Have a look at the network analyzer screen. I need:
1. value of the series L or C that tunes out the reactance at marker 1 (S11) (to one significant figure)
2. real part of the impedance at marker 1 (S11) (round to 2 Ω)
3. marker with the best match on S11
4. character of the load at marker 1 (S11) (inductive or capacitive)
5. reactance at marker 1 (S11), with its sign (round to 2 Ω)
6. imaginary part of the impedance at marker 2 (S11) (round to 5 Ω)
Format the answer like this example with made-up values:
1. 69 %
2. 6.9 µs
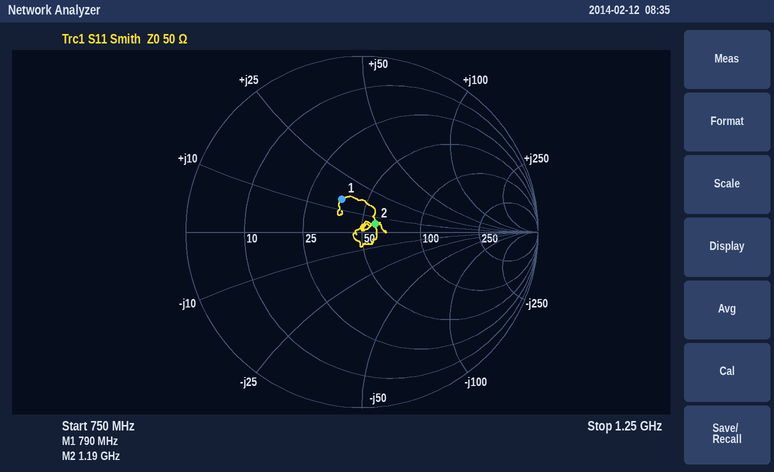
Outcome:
1. 10 pF
2. 38 Ω
3. marker 2
4. inductive
5. +14 Ω
6. +5 Ω
